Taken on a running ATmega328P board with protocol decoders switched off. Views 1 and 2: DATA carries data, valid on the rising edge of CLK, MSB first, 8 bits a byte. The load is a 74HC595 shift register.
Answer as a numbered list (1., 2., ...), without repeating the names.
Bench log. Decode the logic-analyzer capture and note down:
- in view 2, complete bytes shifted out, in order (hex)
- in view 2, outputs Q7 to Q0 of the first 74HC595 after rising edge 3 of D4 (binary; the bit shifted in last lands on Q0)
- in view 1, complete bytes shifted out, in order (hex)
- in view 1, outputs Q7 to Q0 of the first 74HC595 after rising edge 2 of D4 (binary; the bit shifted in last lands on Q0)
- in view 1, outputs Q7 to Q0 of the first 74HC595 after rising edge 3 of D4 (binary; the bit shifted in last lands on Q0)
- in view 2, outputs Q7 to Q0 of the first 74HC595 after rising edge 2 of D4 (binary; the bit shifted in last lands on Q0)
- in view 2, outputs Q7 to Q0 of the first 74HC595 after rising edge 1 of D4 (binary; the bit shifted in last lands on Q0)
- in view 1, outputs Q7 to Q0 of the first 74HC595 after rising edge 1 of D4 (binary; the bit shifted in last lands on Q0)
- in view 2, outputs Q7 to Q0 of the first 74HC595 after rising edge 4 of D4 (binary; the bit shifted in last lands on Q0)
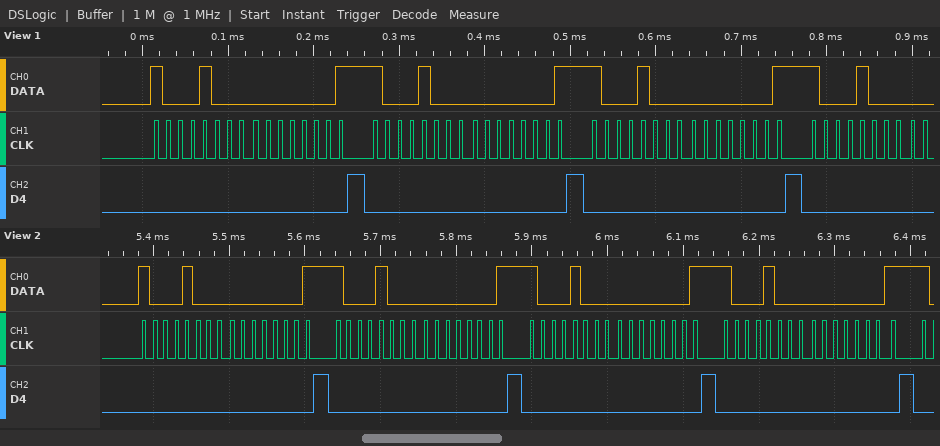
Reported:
1. 0x88 0x01 0x88 0x01 0x88 0x01 0x88 0x01
2. 00000001
3. 0x88 0x01 0x88 0x01 0x88 0x01 0x88
4. 00000001
5. 00000001
6. 00000001
7. 00000001
8. 00000001
9. 00000001
